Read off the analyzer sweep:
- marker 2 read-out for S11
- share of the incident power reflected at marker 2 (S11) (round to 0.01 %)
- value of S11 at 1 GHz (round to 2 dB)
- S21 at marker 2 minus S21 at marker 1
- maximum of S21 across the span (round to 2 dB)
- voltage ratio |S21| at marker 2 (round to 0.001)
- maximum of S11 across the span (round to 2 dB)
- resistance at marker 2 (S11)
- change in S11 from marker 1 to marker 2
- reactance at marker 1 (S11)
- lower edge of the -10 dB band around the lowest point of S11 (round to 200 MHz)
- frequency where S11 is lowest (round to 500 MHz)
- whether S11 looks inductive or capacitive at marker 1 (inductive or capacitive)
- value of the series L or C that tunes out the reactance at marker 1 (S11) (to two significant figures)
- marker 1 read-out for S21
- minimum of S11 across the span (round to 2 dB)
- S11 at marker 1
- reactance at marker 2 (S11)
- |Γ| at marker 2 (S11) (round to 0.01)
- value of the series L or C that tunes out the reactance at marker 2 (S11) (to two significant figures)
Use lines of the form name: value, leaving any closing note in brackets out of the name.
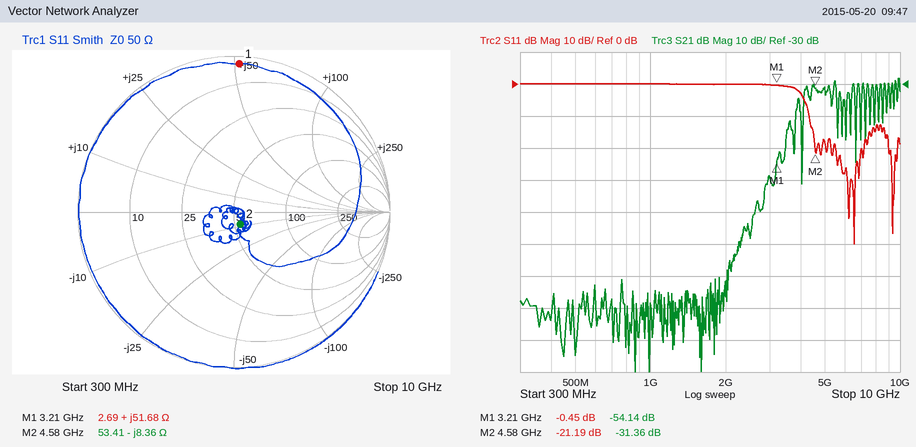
marker 2 read-out for S11: -21.19 dB
share of the incident power reflected at marker 2 (S11): 0.76 %
value of S11 at 1 GHz: 0 dB
S21 at marker 2 minus S21 at marker 1: 22.78 dB
maximum of S21 across the span: -28 dB
voltage ratio |S21| at marker 2: 0.027
maximum of S11 across the span: 0 dB
resistance at marker 2: 53.41 Ω
change in S11 from marker 1 to marker 2: -20.74 dB
reactance at marker 1: +51.68 Ω
lower edge of the -10 dB band around the lowest point of S11: 4.4 GHz
frequency where S11 is lowest: 6.5 GHz
whether S11 looks inductive or capacitive at marker 1: inductive
value of the series L or C that tunes out the reactance at marker 1 (S11): 960 fF
marker 1 read-out for S21: -54.14 dB
minimum of S11 across the span: -50 dB
S11 at marker 1: -0.45 dB
reactance at marker 2: -8.36 Ω
|Γ| at marker 2 (S11): 0.09
value of the series L or C that tunes out the reactance at marker 2 (S11): 290 pH
